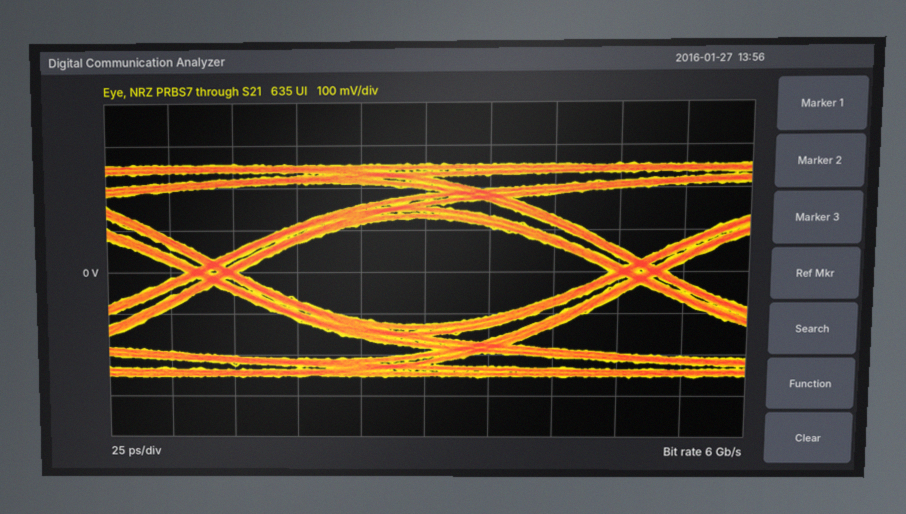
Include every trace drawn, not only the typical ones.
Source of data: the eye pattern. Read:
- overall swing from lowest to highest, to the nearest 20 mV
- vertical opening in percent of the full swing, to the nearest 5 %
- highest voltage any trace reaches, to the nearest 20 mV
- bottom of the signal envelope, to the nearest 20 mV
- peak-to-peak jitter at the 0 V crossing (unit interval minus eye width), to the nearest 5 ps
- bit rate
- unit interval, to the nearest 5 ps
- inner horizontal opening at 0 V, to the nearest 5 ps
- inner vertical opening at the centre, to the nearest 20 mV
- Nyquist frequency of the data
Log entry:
520 mV
50 %
260 mV
-260 mV
20 ps
6 Gb/s
165 ps
145 ps
260 mV
3 GHz
